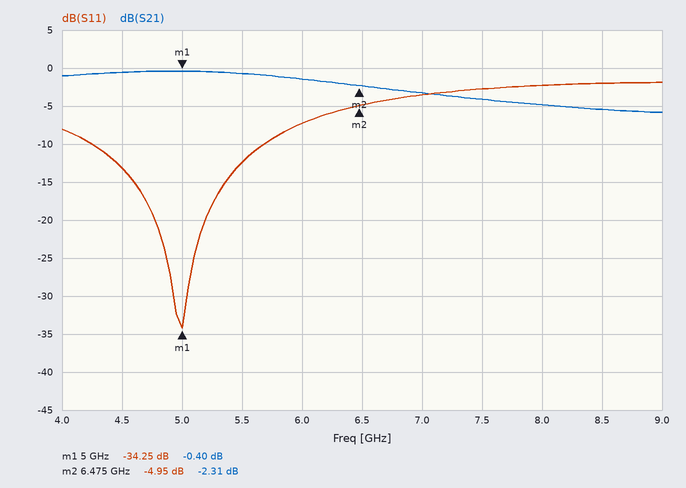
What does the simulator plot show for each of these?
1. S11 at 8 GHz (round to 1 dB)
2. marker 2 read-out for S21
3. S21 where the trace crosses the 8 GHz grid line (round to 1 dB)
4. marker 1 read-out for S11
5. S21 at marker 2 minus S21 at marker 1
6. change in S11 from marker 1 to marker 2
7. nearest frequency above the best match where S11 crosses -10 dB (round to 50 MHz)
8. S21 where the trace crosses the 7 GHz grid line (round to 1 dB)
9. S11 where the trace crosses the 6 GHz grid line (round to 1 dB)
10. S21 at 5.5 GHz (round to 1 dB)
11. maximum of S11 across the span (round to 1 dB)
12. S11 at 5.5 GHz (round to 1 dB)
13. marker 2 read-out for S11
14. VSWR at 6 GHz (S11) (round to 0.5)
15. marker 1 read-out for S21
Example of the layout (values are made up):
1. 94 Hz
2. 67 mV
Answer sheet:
1. -2 dB
2. -2.31 dB
3. -5 dB
4. -34.25 dB
5. -1.91 dB
6. 29.30 dB
7. 5.70 GHz
8. -3 dB
9. -7 dB
10. -1 dB
11. -2 dB
12. -12 dB
13. -4.95 dB
14. 2.5
15. -0.40 dB
